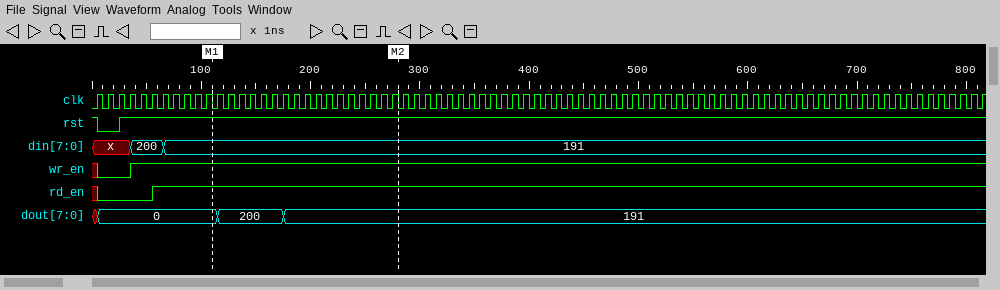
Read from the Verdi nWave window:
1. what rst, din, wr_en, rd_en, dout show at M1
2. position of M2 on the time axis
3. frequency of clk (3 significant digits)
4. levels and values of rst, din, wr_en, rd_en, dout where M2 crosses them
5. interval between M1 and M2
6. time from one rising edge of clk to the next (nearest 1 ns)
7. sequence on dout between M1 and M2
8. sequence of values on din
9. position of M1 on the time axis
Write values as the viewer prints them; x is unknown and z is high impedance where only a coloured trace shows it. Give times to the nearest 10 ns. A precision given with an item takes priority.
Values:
rst=1, din=191, wr_en=1, rd_en=1, dout=0
280 ns
100 MHz
rst=1, din=191, wr_en=1, rd_en=1, dout=191
170 ns
10 ns
0, 200, 191
x, 200, 191
110 ns
